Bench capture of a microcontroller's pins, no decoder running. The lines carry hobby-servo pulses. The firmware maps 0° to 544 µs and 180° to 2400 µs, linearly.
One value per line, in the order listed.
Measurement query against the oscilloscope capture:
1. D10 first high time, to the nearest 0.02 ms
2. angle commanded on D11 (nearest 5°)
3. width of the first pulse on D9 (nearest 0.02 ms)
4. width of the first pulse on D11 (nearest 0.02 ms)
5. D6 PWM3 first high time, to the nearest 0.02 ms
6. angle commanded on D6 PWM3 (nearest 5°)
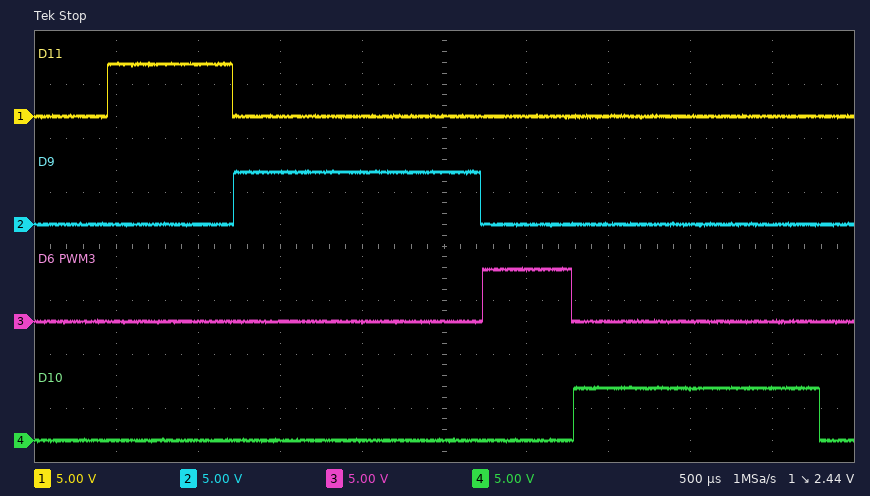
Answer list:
1.50 ms
20°
1.50 ms
0.76 ms
0.54 ms
0°
